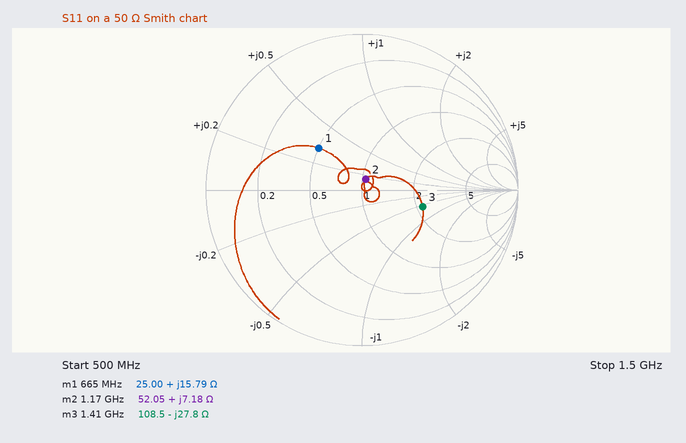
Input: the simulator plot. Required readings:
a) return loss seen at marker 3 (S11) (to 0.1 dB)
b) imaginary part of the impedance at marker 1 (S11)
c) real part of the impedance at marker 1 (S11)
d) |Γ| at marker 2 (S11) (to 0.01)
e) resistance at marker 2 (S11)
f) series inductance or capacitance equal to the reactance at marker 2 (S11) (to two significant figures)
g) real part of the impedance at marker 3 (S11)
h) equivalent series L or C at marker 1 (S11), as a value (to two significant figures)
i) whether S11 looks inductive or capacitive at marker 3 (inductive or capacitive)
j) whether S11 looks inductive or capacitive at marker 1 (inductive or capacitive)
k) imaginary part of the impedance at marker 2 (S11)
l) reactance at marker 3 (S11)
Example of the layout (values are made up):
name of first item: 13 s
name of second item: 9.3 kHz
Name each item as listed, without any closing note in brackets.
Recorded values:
return loss seen at marker 3 (S11): 7.9 dB
imaginary part of the impedance at marker 1: +15.79 Ω
real part of the impedance at marker 1: 25.00 Ω
|Γ| at marker 2 (S11): 0.07
resistance at marker 2: 52.05 Ω
series inductance or capacitance equal to the reactance at marker 2 (S11): 980 pH
real part of the impedance at marker 3: 108.5 Ω
equivalent series L or C at marker 1 (S11), as a value: 3.8 nH
whether S11 looks inductive or capacitive at marker 3: capacitive
whether S11 looks inductive or capacitive at marker 1: inductive
imaginary part of the impedance at marker 2: +7.18 Ω
reactance at marker 3: -27.8 Ω
